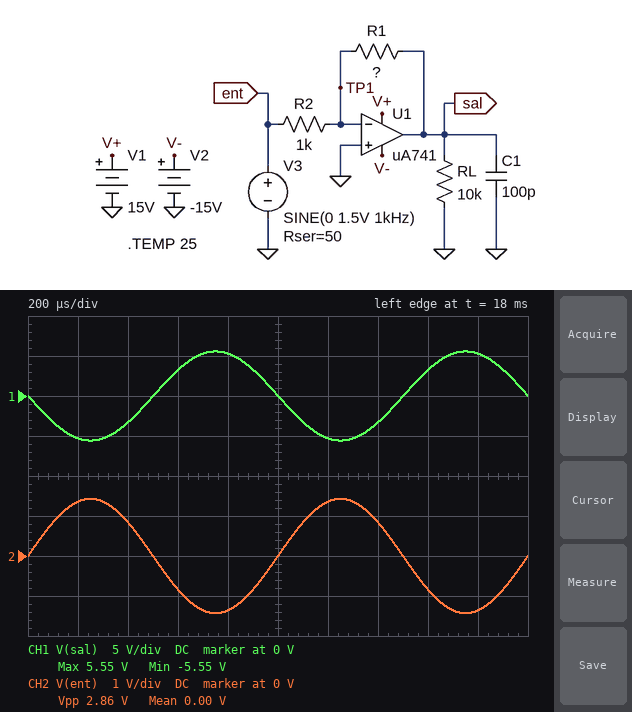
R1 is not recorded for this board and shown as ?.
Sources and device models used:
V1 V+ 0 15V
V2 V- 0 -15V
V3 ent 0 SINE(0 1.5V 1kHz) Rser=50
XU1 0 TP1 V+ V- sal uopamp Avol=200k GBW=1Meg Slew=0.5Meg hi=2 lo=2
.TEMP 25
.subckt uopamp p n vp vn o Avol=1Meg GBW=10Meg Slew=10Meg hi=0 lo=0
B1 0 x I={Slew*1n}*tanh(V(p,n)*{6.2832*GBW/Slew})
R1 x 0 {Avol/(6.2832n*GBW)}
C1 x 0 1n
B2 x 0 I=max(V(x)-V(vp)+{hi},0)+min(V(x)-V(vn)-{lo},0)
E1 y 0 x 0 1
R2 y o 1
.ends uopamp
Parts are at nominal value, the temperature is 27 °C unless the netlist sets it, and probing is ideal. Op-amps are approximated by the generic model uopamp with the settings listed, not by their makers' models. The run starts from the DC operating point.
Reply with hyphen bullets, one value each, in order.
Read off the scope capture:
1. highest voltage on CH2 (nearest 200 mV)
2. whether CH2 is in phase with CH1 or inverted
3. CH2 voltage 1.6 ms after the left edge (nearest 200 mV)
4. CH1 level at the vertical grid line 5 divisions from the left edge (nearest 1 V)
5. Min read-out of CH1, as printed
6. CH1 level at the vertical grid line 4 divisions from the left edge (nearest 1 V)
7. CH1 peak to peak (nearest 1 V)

- 1.4 V
- inverted
- -800 mV
- 0 V
- -5.55 V
- 5 V
- 11 V
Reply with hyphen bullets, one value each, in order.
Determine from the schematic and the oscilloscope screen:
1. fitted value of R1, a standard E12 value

- 3.9 kΩ
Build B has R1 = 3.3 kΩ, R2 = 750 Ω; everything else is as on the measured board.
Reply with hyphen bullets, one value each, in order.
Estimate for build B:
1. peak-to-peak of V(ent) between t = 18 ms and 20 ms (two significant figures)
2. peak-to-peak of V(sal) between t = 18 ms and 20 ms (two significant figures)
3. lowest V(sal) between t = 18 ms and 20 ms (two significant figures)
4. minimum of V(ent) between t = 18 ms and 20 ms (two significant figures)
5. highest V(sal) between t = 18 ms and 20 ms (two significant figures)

- 2.8 V
- 12 V
- -6.2 V
- -1.4 V
- 6.2 V
